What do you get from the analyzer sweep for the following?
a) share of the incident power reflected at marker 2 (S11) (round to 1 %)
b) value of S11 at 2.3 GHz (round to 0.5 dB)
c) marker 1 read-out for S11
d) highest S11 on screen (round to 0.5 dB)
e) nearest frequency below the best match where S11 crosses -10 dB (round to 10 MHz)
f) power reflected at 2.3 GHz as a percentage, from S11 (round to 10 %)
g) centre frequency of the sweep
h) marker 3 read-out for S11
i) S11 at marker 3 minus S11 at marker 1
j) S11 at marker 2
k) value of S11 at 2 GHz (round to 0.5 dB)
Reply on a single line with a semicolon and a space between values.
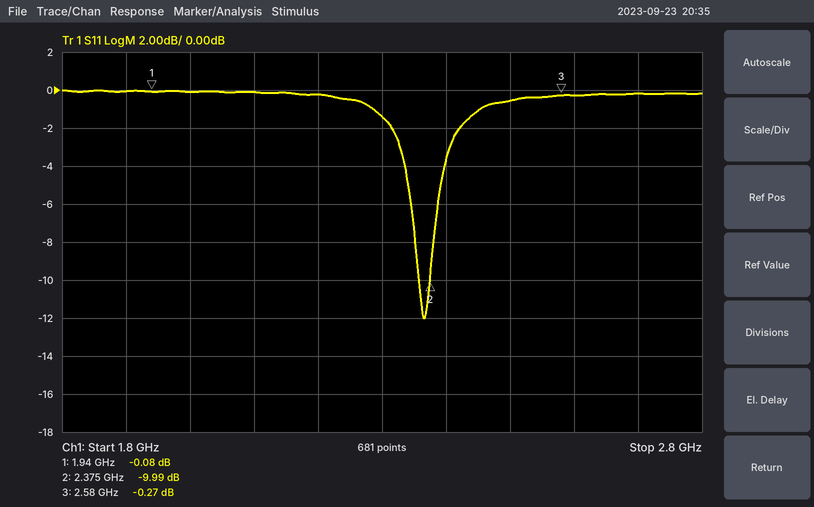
10 %; -1.5 dB; -0.08 dB; 0.0 dB; 2.36 GHz; 70 %; 2.3 GHz; -0.27 dB; -0.19 dB; -9.99 dB; 0.0 dB
